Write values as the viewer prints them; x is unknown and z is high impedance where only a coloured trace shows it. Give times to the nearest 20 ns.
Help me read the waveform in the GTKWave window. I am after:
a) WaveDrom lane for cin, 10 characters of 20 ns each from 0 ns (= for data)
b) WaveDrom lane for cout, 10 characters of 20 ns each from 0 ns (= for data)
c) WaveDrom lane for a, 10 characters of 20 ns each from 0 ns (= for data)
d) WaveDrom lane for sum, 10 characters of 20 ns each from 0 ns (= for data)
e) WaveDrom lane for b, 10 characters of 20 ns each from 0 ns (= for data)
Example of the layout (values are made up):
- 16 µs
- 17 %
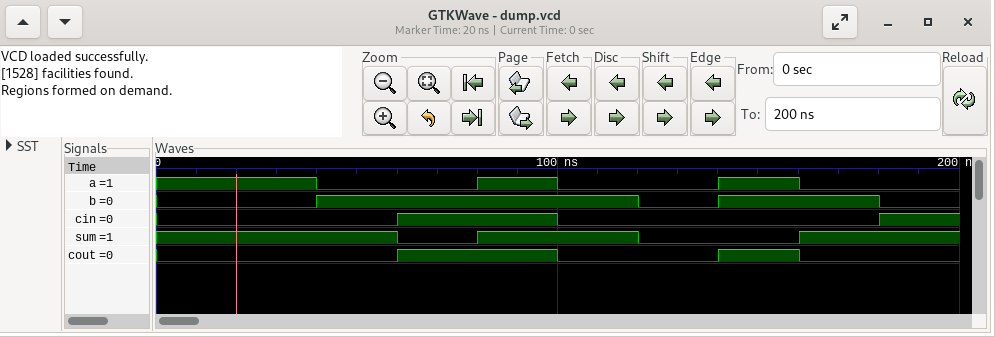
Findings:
- {name: 'cin', wave: '0..1.0...1'}
- {name: 'cout', wave: '0..1.0.10.'}
- {name: 'a', wave: '1.0.10.10.'}
- {name: 'sum', wave: '1..01.0.1.'}
- {name: 'b', wave: '0.1...01.0'}
